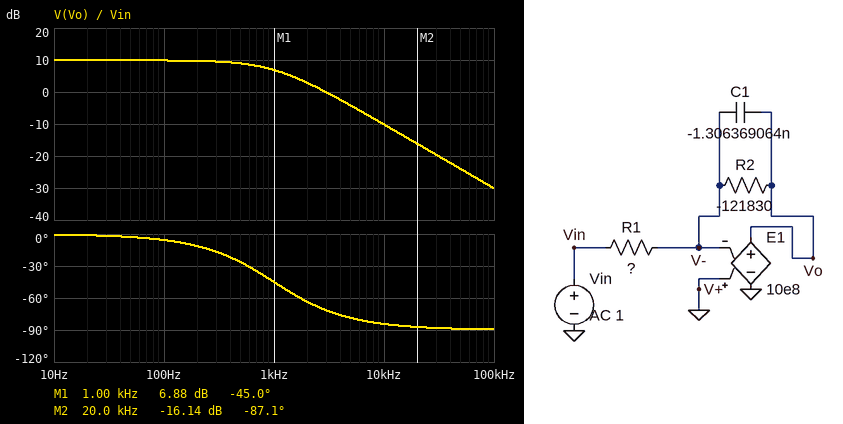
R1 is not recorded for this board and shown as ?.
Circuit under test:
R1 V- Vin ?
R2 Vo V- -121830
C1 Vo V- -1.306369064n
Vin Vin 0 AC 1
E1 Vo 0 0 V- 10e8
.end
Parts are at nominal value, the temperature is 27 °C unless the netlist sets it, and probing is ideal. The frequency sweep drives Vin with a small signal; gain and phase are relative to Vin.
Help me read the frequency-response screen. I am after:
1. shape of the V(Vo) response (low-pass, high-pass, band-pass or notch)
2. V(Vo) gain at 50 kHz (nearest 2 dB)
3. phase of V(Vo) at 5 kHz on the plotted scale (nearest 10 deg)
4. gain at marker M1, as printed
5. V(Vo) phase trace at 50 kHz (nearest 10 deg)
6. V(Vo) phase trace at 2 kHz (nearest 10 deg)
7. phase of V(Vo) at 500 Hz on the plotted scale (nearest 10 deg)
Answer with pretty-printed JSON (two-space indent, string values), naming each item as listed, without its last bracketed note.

{
  "shape of the V(Vo) response": "low-pass",
  "V(Vo) gain at 50 kHz": "-24 dB",
  "phase of V(Vo) at 5 kHz on the plotted scale": "-80 deg",
  "gain at marker M1, as printed": "6.88 dB",
  "V(Vo) phase trace at 50 kHz": "-90 deg",
  "V(Vo) phase trace at 2 kHz": "-60 deg",
  "phase of V(Vo) at 500 Hz on the plotted scale": "-30 deg"
}
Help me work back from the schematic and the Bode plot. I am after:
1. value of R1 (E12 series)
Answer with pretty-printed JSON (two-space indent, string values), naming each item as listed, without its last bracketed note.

{
  "value of R1": "39 kΩ"
}
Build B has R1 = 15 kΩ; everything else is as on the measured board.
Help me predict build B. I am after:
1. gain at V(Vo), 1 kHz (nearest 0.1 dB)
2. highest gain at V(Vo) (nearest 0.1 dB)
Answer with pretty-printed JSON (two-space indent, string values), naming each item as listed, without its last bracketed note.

{
  "gain at V(Vo), 1 kHz": "15.2 dB",
  "highest gain at V(Vo)": "18.2 dB"
}
